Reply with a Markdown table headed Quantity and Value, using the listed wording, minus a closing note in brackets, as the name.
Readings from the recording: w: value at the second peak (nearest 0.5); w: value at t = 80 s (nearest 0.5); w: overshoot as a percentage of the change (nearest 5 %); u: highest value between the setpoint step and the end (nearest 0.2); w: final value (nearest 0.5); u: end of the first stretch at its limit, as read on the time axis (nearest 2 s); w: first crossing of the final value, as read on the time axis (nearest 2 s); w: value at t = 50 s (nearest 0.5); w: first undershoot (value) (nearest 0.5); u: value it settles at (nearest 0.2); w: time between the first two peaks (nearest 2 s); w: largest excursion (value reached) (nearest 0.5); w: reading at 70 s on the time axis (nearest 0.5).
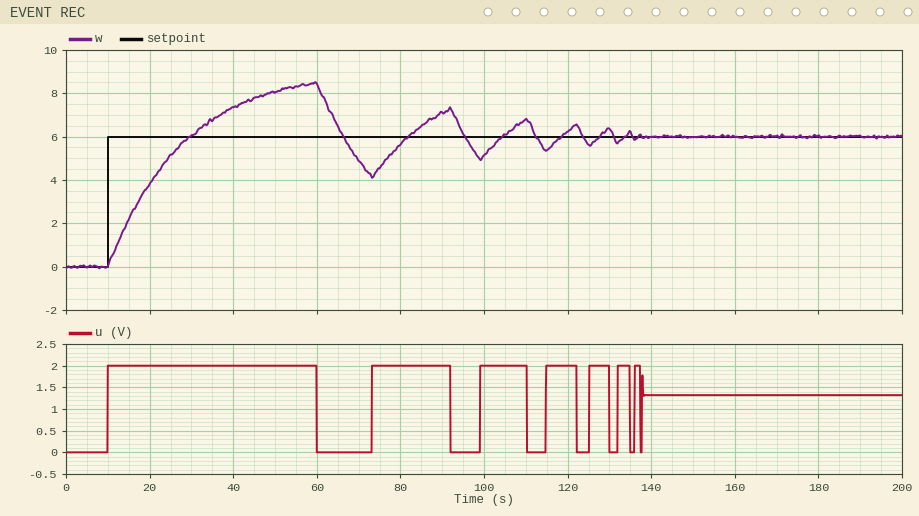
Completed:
| Quantity | Value |
|---|---|
| w: value at the second peak | 7.5 |
| w: value at t = 80 s | 5.5 |
| w: overshoot as a percentage of the change | 40 % |
| u: highest value between the setpoint step and the end | 2.0 |
| w: final value | 6.0 |
| u: end of the first stretch at its limit, as read on the time axis | 60 s |
| w: first crossing of the final value, as read on the time axis | 30 s |
| w: value at t = 50 s | 8.0 |
| w: first undershoot (value) | 4.0 |
| u: value it settles at | 1.4 |
| w: time between the first two peaks | 32 s |
| w: largest excursion (value reached) | 8.5 |
| w: reading at 70 s on the time axis | 5.0 |
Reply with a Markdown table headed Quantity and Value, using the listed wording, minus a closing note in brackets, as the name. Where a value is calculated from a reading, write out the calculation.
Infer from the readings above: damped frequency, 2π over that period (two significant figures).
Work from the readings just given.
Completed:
| Quantity | Value |
|---|---|
| damped frequency, 2π over that period | 2π / 32 = 0.20 rad/s |
